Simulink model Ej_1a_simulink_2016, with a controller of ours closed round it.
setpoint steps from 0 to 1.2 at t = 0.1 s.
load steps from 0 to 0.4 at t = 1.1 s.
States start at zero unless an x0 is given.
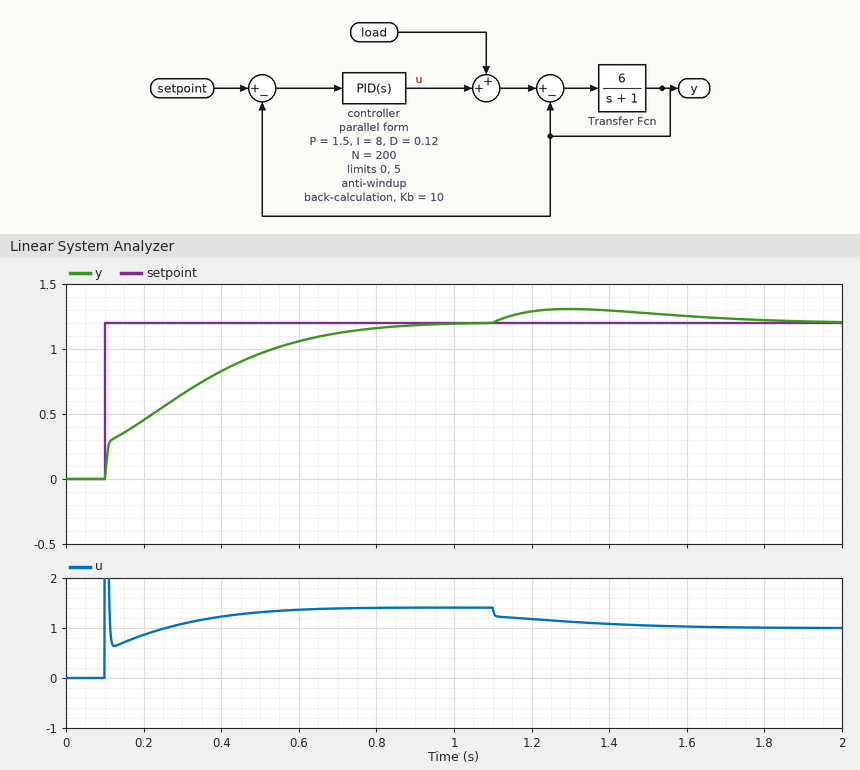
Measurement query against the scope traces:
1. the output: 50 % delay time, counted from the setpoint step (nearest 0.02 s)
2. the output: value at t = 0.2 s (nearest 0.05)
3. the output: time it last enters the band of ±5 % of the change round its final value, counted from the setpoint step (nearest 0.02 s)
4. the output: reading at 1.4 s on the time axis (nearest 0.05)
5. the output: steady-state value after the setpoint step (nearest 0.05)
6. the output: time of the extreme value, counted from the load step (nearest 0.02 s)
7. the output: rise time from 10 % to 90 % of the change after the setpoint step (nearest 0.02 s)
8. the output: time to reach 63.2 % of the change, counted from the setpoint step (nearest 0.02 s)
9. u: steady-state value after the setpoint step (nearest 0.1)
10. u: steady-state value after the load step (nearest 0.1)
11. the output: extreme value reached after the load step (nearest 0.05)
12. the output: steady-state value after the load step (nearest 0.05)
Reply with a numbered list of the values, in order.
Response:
1. 0.18 s
2. 0.45
3. 0.64 s
4. 1.30
5. 1.20
6. 0.20 s
7. 0.52 s
8. 0.26 s
9. 1.4
10. 1.0
11. 1.30
12. 1.20
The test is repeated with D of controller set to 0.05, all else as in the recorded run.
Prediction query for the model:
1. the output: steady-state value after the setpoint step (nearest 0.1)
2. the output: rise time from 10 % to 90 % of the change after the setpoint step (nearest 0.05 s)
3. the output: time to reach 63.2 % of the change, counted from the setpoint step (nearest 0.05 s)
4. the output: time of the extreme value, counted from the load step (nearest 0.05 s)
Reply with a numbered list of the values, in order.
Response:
1. 1.2
2. 0.40 s
3. 0.15 s
4. 0.15 s
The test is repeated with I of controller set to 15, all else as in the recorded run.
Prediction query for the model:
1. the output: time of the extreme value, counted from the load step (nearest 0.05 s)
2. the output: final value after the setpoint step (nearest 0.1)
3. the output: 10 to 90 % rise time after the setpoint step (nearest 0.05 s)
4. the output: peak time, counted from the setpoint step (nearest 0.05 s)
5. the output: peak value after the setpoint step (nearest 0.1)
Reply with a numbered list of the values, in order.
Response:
1. 0.15 s
2. 1.2
3. 0.30 s
4. 0.55 s
5. 1.3
